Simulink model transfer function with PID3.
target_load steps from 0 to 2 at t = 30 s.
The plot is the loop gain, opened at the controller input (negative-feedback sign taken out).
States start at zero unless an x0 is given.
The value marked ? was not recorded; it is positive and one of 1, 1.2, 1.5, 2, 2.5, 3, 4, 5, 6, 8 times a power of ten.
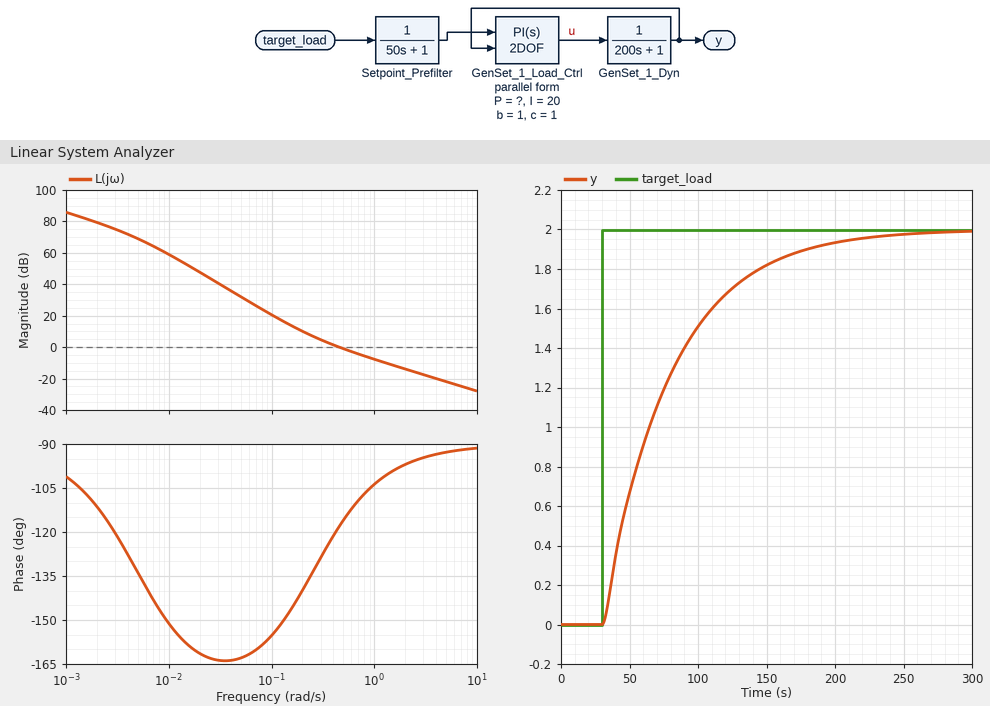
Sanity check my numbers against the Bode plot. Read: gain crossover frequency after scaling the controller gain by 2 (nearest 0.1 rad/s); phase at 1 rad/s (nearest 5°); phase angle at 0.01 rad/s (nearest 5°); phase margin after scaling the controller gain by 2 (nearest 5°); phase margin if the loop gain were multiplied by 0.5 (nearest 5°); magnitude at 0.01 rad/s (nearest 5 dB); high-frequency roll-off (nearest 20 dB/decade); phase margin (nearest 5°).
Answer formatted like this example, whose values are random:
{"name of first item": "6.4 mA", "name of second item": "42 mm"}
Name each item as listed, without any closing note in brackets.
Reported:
{"gain crossover frequency after scaling the controller gain by 2": "0.8 rad/s", "phase at 1 rad/s": "-105°", "phase angle at 0.01 rad/s": "-150°", "phase margin after scaling the controller gain by 2": "75°", "phase margin if the loop gain were multiplied by 0.5": "50°", "magnitude at 0.01 rad/s": "60 dB", "high-frequency roll-off": "-20 dB/decade", "phase margin": "60°"}
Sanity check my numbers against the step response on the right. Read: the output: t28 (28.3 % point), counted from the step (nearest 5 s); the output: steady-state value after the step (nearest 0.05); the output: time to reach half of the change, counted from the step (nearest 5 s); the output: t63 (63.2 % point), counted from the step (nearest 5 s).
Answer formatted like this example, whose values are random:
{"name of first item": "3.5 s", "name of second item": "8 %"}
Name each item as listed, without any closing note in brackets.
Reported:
{"the output: t28 (28.3 % point), counted from the step": "15 s", "the output: steady-state value after the step": "2.00", "the output: time to reach half of the change, counted from the step": "35 s", "the output: t63 (63.2 % point), counted from the step": "50 s"}
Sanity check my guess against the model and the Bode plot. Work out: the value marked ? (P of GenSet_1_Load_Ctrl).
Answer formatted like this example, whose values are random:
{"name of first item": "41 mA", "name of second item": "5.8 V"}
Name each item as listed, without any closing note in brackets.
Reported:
{"the value marked ?": "80"}
